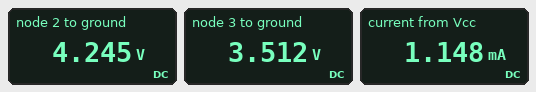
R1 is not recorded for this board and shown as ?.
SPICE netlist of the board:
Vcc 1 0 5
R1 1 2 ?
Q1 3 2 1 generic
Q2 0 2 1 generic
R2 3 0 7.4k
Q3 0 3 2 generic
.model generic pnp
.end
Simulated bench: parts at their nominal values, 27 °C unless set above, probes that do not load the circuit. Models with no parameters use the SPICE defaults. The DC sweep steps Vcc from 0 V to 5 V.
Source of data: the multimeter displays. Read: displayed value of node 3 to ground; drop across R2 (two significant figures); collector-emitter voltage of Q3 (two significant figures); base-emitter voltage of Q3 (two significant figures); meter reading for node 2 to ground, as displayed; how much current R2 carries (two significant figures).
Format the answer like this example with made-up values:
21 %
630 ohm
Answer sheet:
3.512 V
3.5 V
-4.2 V
-730 mV
4.245 V
470 µA
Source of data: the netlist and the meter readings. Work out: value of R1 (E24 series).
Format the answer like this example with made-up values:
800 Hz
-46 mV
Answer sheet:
3.9 kΩ
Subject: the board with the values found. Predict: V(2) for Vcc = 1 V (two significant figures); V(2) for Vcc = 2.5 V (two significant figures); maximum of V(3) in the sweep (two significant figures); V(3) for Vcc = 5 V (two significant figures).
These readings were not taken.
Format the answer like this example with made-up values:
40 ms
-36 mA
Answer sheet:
710 mV
1.8 V
3.5 V
3.5 V
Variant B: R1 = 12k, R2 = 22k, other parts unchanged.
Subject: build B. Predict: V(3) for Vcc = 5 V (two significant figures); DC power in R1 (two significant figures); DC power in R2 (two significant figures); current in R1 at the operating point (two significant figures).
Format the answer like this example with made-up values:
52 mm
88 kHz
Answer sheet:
3.6 V
44 µW
580 µW
61 µA
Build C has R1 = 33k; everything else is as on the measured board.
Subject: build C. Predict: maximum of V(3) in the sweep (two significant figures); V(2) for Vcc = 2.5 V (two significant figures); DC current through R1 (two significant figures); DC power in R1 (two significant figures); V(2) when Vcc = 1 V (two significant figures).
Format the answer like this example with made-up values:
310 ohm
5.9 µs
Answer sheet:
3.6 V
1.8 V
23 µA
17 µW
660 mV
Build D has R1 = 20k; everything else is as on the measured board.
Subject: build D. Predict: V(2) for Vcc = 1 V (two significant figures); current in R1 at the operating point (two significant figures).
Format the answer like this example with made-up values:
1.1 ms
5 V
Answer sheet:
670 mV
38 µA
